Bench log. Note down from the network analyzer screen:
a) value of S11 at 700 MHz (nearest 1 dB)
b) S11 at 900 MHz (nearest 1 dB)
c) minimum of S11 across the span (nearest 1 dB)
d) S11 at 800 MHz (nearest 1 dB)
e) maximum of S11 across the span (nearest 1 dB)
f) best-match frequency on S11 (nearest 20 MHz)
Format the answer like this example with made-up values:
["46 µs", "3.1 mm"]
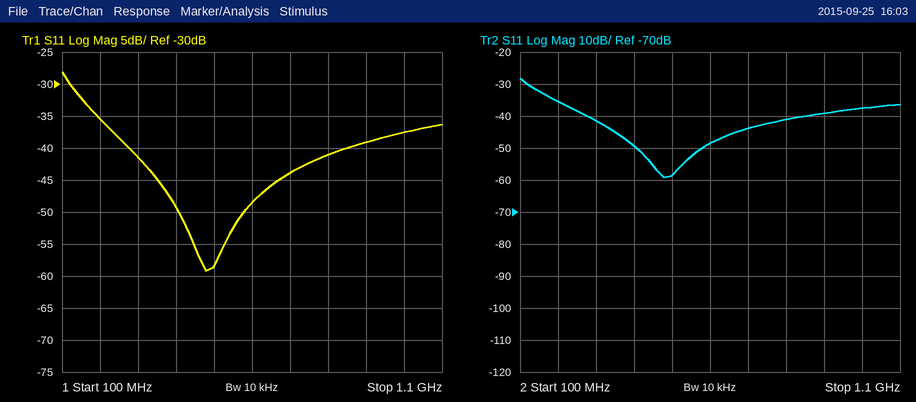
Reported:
["-44 dB", "-39 dB", "-59 dB", "-41 dB", "-28 dB", "480 MHz"]
